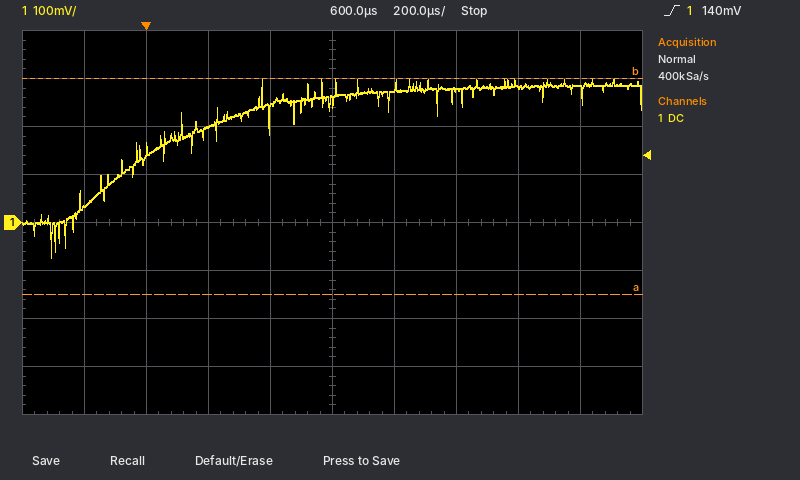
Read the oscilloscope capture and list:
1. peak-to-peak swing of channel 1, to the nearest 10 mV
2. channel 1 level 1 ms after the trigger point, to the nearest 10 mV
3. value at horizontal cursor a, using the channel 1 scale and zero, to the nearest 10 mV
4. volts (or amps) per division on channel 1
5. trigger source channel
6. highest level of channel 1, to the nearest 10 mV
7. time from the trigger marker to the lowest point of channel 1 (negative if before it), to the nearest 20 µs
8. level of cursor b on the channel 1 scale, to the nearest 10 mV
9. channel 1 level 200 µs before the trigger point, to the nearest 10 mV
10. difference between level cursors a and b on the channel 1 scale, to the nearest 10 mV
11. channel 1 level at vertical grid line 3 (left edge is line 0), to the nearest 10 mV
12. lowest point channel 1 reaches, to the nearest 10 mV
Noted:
370 mV
280 mV
-150 mV
100 mV
channel 1
300 mV
-300 µs
300 mV
30 mV
450 mV
200 mV
-70 mV
